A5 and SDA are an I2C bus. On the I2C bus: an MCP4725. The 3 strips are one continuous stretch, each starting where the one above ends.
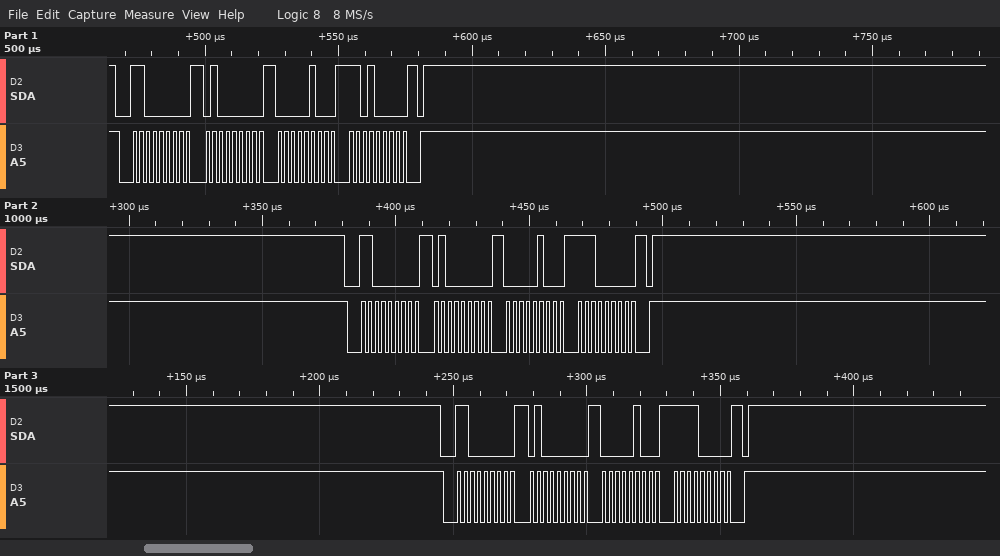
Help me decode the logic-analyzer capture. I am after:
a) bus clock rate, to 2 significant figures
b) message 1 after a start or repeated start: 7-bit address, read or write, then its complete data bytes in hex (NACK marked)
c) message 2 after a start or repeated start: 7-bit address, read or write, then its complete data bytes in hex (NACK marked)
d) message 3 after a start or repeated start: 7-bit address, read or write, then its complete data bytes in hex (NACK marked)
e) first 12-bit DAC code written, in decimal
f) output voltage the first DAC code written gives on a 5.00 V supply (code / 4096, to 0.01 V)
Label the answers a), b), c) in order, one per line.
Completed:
a) 400 kHz
b) 0x60 write: 40 04 D0
c) 0x60 write: 40 04 E0
d) 0x60 write: 40 04 F0
e) 77
f) 0.09 V
